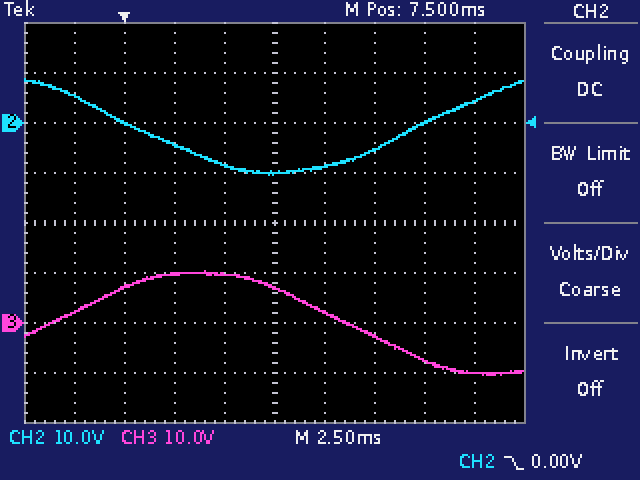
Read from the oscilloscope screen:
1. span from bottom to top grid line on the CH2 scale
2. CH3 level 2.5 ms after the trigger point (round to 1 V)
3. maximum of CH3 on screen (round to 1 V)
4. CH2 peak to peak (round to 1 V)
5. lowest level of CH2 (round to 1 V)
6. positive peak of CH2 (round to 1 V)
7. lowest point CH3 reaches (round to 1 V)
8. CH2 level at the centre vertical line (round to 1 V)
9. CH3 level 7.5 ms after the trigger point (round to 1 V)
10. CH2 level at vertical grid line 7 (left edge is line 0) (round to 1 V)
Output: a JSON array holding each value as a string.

["80 V", "10 V", "10 V", "19 V", "-10 V", "9 V", "-10 V", "-10 V", "7 V", "-5 V"]
